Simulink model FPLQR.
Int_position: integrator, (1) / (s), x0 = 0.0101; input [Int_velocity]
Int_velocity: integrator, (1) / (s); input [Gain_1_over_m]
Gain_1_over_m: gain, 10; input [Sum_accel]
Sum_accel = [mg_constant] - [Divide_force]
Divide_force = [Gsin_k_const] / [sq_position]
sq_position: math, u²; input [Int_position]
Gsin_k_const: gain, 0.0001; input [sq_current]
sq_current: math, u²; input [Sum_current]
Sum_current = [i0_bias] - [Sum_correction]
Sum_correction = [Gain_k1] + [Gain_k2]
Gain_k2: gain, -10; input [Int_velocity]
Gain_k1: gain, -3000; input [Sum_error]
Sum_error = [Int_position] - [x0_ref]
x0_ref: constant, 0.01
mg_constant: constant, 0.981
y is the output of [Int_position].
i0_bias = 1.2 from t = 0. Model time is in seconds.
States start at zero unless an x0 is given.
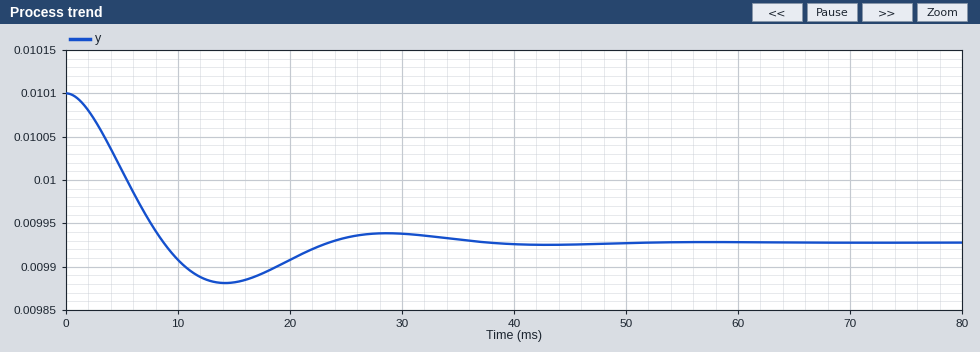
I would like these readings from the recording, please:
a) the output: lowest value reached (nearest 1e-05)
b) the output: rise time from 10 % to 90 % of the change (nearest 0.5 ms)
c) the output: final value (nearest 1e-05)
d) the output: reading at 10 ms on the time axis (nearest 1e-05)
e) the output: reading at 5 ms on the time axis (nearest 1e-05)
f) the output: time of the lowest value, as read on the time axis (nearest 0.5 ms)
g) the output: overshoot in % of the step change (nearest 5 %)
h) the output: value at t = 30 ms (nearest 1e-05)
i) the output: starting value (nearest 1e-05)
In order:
0.00988
6.0 ms
0.00993
0.00991
0.01001
14.0 ms
25 %
0.00994
0.01010
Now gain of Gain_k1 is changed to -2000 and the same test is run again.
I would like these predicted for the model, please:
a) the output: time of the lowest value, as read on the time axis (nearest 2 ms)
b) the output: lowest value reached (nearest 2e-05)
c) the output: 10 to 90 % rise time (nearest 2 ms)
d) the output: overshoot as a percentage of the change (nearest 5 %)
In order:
18 ms
0.00986
8 ms
15 %
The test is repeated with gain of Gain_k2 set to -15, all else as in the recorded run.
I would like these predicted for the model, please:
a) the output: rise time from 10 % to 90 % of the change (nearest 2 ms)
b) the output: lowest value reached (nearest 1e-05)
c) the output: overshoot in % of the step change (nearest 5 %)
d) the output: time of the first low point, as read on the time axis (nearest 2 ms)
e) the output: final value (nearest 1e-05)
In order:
8 ms
0.00991
10 %
16 ms
0.00993
